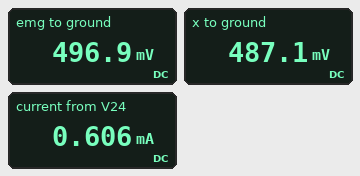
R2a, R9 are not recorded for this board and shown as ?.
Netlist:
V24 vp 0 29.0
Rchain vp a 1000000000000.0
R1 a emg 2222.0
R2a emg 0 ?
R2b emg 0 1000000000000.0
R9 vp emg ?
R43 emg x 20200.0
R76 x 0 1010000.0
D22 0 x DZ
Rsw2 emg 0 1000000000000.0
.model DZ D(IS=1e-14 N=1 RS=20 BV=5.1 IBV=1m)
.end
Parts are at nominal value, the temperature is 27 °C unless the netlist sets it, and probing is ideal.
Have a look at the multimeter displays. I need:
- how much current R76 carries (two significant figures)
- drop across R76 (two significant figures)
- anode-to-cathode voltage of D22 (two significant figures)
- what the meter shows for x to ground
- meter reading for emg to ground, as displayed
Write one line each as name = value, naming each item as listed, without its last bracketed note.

how much current R76 carries = 480 nA
drop across R76 = 490 mV
anode-to-cathode voltage of D22 = -490 mV
what the meter shows for x to ground = 487.1 mV
meter reading for emg to ground, as displayed = 496.9 mV
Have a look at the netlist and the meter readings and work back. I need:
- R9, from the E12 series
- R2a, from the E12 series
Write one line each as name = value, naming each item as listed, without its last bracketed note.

R9, from the E12 series = 47 kΩ
R2a, from the E12 series = 820 Ω
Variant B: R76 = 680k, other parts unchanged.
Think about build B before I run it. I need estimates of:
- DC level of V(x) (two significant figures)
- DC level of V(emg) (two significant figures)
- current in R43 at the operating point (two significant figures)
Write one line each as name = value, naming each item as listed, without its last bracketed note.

DC level of V(x) = 480 mV
DC level of V(emg) = 500 mV
current in R43 at the operating point = 710 nA
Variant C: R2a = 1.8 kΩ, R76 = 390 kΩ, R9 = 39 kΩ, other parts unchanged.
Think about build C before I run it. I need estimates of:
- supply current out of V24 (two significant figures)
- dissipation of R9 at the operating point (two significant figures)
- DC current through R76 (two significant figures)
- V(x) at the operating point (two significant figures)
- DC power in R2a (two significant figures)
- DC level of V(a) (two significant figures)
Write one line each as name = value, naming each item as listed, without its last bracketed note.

supply current out of V24 = 710 µA
dissipation of R9 at the operating point = 20 mW
DC current through R76 = 3.1 µA
V(x) at the operating point = 1.2 V
DC power in R2a = 900 µW
DC level of V(a) = 1.3 V
